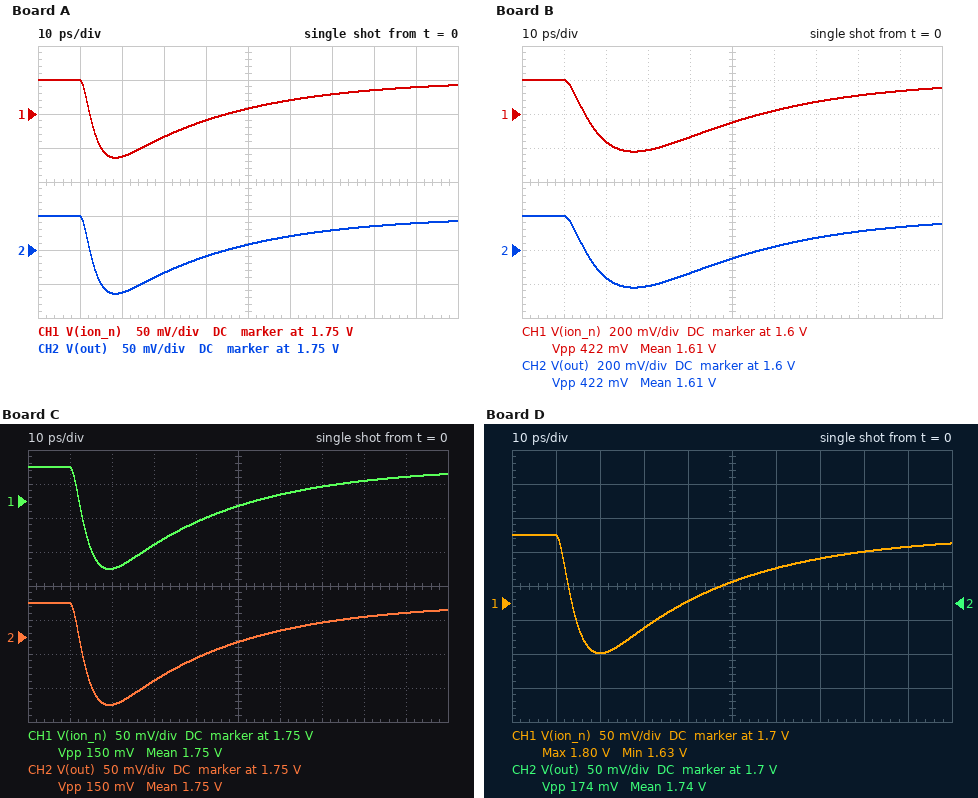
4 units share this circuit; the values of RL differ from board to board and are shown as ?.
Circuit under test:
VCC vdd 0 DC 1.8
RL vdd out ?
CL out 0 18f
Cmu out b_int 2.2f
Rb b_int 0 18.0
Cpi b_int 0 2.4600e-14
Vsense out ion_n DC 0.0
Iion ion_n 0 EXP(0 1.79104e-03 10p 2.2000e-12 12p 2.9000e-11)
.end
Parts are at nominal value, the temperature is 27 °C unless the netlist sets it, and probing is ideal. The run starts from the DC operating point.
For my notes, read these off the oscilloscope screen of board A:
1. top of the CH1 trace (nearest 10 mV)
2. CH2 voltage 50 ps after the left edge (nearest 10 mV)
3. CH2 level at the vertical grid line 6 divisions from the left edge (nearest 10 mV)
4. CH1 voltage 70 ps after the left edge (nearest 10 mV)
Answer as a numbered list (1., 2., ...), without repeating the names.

1. 1.80 V
2. 1.76 V
3. 1.77 V
4. 1.78 V
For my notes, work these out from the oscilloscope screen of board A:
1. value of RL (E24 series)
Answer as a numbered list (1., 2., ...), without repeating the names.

1. 82 Ω
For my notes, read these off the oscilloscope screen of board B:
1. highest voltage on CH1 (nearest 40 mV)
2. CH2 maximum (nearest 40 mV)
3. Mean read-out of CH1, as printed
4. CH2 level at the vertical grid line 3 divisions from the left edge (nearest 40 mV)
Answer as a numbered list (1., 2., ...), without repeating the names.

1. 1.80 V
2. 1.80 V
3. 1.61 V
4. 1.40 V
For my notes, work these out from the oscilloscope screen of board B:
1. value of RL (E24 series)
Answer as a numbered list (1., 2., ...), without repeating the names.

1. 390 Ω
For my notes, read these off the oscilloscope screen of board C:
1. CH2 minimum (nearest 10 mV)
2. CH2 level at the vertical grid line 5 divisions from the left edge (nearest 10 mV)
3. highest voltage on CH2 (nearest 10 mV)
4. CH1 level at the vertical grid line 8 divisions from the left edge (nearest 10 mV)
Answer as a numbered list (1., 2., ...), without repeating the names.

1. 1.65 V
2. 1.74 V
3. 1.80 V
4. 1.78 V
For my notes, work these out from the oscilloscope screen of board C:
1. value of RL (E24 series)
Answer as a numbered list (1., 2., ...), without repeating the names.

1. 110 Ω
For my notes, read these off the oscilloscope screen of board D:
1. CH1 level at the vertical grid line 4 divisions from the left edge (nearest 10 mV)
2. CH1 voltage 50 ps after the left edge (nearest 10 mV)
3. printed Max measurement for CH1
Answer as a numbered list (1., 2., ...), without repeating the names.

1. 1.70 V
2. 1.73 V
3. 1.80 V
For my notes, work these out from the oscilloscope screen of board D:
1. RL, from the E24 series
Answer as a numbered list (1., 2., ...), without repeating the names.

1. 130 Ω
